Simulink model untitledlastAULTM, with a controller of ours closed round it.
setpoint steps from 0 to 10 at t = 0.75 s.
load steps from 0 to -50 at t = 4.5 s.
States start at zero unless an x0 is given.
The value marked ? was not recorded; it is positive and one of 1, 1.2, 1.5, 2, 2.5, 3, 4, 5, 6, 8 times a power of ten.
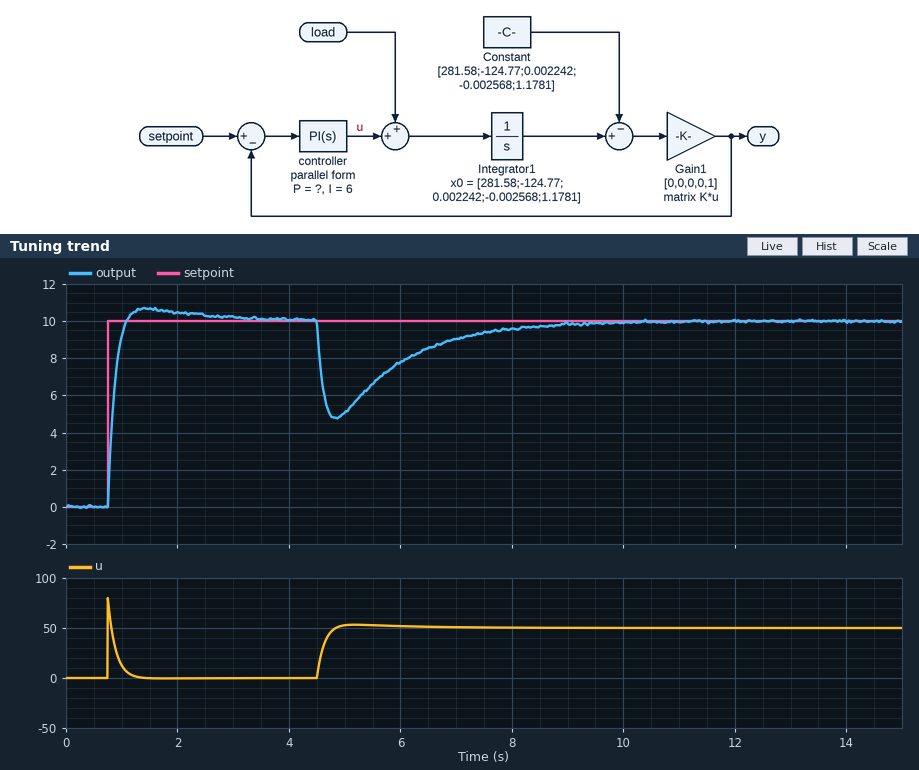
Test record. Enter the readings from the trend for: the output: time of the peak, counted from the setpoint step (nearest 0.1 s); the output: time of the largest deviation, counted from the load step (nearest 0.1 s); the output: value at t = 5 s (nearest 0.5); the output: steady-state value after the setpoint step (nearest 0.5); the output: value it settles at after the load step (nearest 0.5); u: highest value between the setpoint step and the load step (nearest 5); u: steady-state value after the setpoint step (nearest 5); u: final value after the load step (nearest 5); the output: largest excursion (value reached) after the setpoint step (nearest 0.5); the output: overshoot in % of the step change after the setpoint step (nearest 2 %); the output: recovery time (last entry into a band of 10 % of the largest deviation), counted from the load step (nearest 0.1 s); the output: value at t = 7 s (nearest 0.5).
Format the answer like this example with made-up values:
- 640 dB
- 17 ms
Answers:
- 0.7 s
- 0.3 s
- 5.0
- 10.0
- 10.0
- 80
- 0
- 50
- 10.5
- 6 %
- 3.2 s
- 9.0
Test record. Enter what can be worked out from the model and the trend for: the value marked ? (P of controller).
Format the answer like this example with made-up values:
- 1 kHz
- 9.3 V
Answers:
- 8
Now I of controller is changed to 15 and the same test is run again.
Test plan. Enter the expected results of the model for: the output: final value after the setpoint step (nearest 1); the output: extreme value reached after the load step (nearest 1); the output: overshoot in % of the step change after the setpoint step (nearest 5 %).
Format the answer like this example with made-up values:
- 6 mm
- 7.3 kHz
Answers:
- 10
- 5
- 15 %
